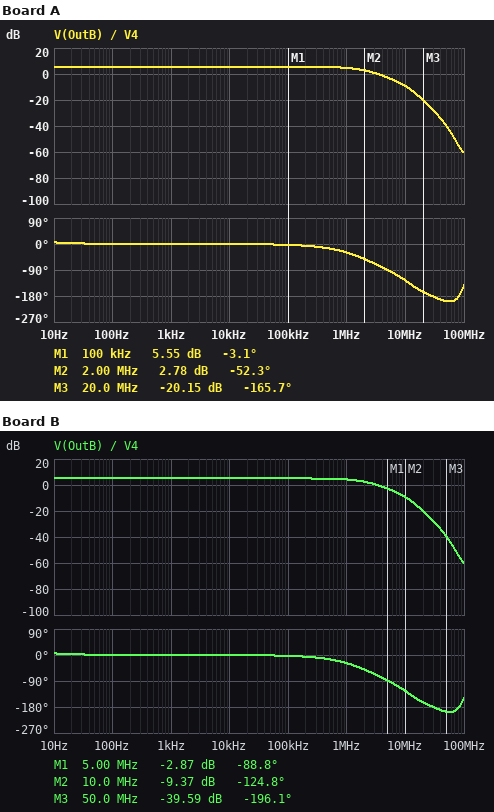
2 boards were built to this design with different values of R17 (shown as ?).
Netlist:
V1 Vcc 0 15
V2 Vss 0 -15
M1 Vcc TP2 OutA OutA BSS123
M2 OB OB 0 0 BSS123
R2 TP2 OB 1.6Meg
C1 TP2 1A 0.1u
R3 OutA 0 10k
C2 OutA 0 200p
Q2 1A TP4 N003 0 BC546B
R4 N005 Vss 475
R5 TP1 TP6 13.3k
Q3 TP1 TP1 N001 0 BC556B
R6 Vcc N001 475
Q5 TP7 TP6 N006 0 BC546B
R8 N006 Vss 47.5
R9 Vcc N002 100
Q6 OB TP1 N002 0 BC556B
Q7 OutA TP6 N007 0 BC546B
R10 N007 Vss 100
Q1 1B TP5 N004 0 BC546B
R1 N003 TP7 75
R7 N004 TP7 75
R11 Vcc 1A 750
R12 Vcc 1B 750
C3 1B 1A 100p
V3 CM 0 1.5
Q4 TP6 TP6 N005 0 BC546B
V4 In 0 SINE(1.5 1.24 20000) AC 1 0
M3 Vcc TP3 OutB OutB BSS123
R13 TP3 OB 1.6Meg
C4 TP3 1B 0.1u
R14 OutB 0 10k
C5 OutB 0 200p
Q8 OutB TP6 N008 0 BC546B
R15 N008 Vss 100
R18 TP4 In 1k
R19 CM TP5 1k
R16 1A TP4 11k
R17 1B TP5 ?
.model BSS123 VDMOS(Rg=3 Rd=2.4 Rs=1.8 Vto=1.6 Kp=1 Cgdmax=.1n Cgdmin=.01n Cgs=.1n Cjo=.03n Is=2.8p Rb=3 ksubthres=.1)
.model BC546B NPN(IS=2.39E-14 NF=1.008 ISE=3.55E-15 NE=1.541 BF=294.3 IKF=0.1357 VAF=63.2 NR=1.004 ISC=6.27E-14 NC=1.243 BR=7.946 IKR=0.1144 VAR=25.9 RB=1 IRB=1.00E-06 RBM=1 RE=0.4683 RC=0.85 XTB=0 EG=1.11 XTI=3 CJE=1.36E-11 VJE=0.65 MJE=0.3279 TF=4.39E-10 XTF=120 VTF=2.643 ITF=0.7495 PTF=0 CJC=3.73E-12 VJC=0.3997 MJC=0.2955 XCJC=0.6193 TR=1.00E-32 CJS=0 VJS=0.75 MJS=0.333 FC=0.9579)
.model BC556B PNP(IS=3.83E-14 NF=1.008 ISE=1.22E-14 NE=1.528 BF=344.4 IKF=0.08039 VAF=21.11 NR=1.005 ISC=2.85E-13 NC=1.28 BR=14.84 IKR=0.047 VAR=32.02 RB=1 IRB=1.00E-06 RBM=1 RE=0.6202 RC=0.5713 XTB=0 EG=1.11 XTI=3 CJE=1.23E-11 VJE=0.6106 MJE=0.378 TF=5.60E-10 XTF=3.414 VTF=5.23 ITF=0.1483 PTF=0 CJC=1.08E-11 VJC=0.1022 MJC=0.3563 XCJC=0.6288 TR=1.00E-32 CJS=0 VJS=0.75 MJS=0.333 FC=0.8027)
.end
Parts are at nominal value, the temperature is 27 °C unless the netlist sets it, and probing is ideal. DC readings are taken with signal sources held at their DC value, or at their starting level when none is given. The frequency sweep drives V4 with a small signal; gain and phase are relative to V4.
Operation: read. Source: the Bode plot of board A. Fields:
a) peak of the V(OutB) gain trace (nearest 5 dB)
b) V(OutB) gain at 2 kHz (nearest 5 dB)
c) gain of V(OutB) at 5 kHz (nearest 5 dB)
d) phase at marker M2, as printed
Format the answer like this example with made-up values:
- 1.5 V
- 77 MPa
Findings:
- 5 dB
- 5 dB
- 5 dB
- -52.3 deg
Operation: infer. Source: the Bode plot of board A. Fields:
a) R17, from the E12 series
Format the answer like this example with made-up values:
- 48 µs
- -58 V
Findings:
- 5.6 kΩ
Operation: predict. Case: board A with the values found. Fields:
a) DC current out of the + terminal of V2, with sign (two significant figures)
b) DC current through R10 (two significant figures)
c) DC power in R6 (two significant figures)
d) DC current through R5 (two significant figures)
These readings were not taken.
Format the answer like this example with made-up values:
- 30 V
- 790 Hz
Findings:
- -37 mA
- 8.7 mA
- 1.9 mW
- 2.0 mA
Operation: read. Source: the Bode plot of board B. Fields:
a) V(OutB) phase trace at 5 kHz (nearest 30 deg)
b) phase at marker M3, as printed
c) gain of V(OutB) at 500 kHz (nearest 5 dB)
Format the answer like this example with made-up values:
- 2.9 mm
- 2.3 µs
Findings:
- 0 deg
- -196.1 deg
- 5 dB
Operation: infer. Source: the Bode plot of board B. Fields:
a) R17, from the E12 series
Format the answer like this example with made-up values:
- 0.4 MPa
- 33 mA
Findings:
- 4.7 kΩ
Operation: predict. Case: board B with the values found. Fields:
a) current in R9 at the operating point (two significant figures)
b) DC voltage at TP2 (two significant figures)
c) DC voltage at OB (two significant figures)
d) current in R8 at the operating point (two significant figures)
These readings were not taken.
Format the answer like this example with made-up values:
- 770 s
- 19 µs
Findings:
- 9.2 mA
- 1.7 V
- 1.7 V
- 18 mA
